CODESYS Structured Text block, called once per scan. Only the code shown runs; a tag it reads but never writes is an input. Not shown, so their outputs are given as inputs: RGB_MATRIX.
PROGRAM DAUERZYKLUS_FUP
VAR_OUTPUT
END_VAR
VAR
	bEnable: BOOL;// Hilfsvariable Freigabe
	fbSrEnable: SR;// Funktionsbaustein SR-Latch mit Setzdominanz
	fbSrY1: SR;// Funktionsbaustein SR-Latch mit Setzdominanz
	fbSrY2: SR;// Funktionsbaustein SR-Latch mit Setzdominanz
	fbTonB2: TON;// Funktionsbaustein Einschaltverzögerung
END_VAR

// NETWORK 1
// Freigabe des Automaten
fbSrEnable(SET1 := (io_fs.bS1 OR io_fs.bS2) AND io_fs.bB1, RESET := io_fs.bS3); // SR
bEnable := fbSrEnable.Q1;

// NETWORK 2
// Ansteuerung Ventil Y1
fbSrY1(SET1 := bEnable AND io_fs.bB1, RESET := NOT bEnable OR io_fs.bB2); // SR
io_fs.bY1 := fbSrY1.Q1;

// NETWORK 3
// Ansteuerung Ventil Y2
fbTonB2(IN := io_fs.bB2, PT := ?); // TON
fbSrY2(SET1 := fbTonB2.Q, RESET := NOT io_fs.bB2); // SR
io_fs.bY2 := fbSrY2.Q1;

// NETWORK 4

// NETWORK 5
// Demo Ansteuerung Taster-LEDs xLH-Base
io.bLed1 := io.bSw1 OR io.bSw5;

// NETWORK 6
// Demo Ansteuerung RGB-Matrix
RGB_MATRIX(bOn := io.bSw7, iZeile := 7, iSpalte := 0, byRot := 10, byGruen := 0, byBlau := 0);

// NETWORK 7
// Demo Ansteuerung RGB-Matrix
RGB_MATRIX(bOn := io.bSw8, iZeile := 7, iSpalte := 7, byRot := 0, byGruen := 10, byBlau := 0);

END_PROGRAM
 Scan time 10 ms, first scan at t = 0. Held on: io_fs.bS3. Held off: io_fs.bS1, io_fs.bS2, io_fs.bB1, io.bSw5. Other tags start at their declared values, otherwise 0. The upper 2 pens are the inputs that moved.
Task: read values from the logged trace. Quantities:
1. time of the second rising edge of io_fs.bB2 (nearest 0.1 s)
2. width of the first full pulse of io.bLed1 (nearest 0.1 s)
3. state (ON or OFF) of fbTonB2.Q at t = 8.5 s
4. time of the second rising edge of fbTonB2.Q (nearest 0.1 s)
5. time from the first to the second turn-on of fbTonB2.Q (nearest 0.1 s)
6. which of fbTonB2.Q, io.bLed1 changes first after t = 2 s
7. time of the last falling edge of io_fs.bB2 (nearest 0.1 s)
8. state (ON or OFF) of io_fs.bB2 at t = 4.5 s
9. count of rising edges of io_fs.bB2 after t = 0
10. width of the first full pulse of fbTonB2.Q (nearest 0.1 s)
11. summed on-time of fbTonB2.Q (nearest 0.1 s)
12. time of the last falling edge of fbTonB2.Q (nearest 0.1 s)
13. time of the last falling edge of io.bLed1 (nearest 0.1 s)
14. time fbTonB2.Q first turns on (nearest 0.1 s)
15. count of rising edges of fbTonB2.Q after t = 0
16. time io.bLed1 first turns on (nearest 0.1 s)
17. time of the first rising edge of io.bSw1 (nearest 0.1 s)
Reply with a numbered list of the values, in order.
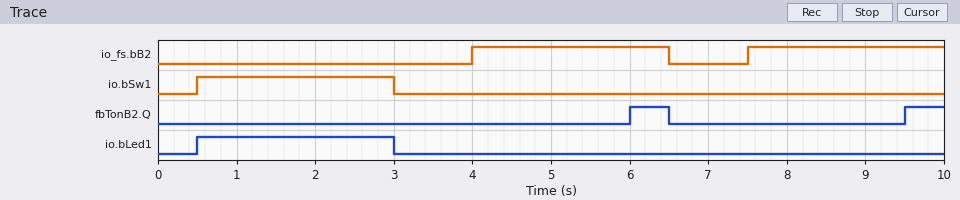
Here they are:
1. 7.5 s
2. 2.5 s
3. OFF
4. 9.5 s
5. 3.5 s
6. io.bLed1
7. 6.5 s
8. ON
9. 2
10. 0.5 s
11. 1.0 s
12. 6.5 s
13. 3.0 s
14. 6.0 s
15. 2
16. 0.5 s
17. 0.5 s
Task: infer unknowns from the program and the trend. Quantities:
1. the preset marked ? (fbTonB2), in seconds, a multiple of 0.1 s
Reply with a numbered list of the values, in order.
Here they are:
1. 2.0 s
